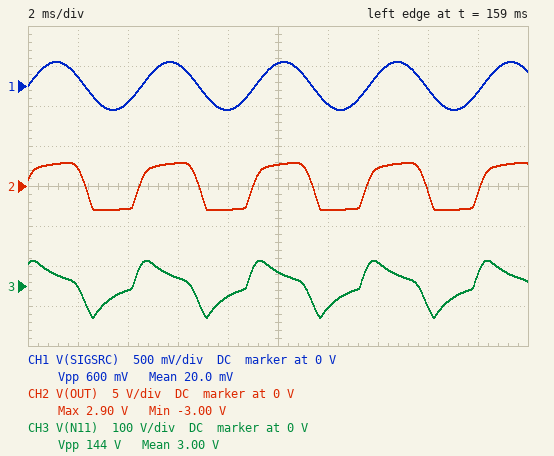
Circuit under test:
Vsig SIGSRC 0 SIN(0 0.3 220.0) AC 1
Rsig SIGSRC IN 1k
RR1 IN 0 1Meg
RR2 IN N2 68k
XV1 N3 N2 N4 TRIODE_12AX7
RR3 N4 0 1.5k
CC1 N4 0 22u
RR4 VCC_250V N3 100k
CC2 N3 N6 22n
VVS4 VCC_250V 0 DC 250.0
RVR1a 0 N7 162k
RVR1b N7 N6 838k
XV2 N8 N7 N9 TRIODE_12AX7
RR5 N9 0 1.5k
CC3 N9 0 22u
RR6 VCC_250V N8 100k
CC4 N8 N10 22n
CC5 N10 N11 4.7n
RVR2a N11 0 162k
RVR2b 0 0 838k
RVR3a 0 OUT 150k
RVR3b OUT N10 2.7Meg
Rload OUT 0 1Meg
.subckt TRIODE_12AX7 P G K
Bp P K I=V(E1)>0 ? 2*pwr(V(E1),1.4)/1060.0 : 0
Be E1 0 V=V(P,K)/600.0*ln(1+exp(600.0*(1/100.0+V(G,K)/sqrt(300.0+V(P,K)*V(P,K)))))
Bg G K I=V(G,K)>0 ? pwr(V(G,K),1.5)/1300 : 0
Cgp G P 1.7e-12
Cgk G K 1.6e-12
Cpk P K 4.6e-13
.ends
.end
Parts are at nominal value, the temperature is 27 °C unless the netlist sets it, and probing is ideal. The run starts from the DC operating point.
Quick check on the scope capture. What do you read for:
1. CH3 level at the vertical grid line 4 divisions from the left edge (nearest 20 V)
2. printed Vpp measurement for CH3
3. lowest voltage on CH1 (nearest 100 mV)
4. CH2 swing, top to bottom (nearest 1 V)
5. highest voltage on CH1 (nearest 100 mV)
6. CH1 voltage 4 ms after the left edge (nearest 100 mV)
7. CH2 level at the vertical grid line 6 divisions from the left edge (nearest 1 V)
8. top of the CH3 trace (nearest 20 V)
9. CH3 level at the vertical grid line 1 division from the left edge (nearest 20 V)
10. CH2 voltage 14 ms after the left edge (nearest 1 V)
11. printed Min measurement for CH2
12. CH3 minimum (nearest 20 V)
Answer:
-20 V
144 V
-300 mV
6 V
300 mV
-200 mV
-3 V
60 V
0 V
2 V
-3.00 V
-80 V
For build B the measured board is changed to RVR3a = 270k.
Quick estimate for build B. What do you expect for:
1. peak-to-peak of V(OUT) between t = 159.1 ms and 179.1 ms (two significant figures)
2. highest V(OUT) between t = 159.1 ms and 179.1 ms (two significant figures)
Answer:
9.3 V
4.6 V
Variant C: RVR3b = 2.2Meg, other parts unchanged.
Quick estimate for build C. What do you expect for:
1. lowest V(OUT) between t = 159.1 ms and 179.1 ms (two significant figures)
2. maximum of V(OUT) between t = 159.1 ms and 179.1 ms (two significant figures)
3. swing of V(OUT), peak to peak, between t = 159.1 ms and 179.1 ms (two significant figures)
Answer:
-3.6 V
3.5 V
7.1 V
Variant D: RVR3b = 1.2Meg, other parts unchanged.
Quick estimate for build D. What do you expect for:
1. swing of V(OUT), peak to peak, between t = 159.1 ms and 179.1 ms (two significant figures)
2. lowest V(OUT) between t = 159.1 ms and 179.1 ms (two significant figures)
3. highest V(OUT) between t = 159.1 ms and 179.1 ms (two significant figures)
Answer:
12 V
-6.3 V
6.0 V
